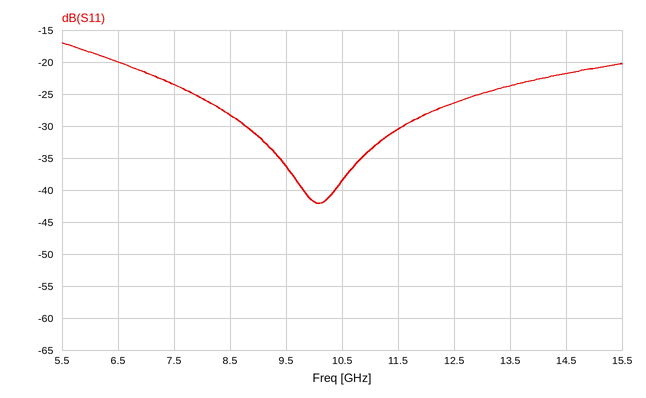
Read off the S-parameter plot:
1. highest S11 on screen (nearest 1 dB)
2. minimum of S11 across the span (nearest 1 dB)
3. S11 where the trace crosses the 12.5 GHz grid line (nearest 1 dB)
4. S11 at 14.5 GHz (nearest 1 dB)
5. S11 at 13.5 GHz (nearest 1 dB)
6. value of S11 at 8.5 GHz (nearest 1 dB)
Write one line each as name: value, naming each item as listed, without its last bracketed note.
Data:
highest S11 on screen: -17 dB
minimum of S11 across the span: -42 dB
S11 where the trace crosses the 12.5 GHz grid line: -26 dB
S11 at 14.5 GHz: -22 dB
S11 at 13.5 GHz: -24 dB
value of S11 at 8.5 GHz: -28 dB
